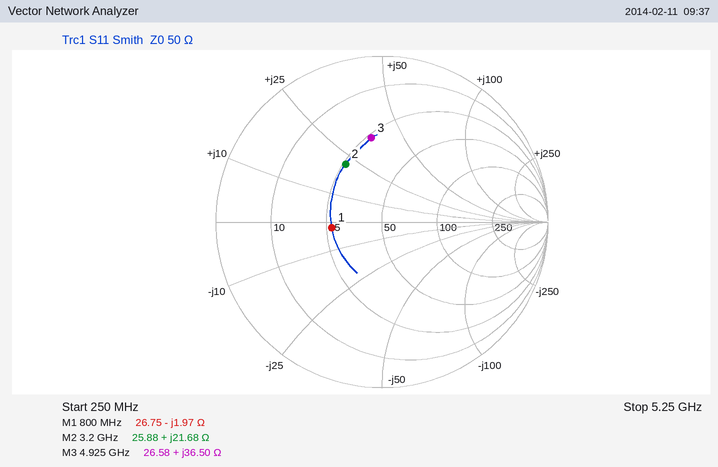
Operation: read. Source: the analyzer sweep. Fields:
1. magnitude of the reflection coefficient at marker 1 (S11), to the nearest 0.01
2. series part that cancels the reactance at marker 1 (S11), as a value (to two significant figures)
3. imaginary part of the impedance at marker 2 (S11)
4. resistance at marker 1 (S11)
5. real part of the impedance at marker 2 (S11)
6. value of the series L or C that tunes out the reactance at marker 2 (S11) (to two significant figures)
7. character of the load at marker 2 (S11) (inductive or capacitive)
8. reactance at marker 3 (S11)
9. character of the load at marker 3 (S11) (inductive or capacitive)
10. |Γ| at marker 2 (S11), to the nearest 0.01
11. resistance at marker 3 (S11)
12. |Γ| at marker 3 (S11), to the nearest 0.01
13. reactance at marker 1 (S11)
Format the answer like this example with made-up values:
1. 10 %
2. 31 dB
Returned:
1. 0.30
2. 390 pH
3. +21.68 Ω
4. 26.75 Ω
5. 25.88 Ω
6. 2.3 pF
7. inductive
8. +36.50 Ω
9. inductive
10. 0.41
11. 26.58 Ω
12. 0.51
13. -1.97 Ω
